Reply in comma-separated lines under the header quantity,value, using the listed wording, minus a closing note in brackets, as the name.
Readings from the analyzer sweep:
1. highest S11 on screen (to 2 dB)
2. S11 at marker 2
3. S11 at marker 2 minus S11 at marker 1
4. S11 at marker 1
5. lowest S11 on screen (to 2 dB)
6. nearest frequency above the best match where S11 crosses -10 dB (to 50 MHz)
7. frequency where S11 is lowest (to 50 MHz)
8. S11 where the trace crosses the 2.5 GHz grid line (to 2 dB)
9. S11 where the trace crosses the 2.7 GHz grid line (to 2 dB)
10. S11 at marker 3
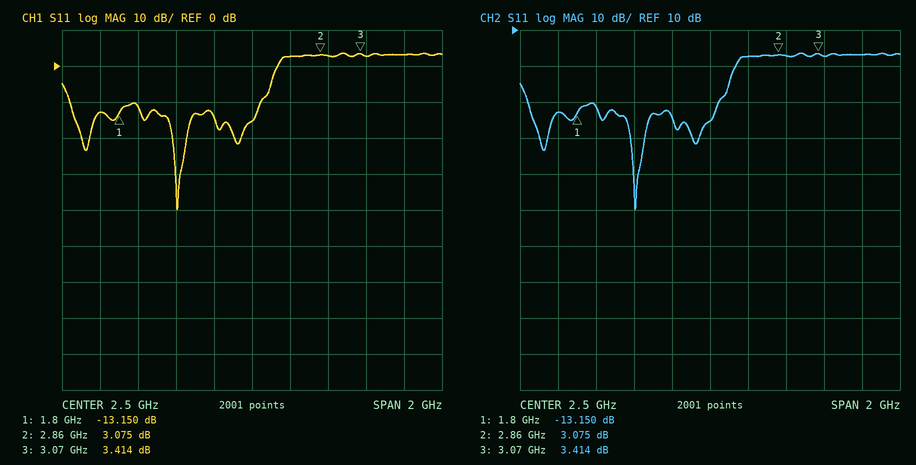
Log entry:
quantity,value
highest S11 on screen,4 dB
S11 at marker 2,3.075 dB
S11 at marker 2 minus S11 at marker 1,16.225 dB
S11 at marker 1,-13.150 dB
lowest S11 on screen,-40 dB
nearest frequency above the best match where S11 crosses -10 dB,2.55 GHz
frequency where S11 is lowest,2.10 GHz
S11 where the trace crosses the 2.5 GHz grid line,-16 dB
S11 where the trace crosses the 2.7 GHz grid line,2 dB
S11 at marker 3,3.414 dB
